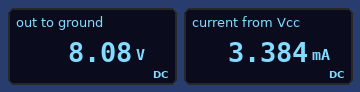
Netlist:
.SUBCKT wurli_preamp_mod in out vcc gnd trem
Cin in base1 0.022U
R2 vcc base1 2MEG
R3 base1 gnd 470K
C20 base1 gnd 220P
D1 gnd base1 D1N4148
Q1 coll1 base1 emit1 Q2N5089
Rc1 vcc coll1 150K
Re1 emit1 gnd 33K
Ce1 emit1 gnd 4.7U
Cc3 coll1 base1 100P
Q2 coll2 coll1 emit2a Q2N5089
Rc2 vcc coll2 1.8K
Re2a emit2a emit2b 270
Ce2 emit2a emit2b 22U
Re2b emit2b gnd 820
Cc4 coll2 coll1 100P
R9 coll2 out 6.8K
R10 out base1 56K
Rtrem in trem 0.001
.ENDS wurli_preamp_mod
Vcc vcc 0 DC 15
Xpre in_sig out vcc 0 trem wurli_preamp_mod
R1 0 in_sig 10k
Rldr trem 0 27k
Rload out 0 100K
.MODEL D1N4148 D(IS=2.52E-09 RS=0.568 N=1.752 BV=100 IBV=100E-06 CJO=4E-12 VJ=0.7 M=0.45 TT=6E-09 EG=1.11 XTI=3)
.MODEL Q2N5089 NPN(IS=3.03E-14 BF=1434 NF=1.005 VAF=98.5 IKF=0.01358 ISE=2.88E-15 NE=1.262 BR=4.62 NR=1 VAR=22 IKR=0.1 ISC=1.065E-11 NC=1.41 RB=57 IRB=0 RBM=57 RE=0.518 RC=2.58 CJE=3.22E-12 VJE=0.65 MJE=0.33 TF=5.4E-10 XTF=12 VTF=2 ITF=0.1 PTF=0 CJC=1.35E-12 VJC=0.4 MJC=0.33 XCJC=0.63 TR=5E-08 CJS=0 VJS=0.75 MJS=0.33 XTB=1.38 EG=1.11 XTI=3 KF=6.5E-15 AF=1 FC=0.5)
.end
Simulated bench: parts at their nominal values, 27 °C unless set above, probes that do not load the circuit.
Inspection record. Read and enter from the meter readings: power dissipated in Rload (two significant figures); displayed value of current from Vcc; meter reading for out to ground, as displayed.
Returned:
650 µW
3.384 mA
8.08 V
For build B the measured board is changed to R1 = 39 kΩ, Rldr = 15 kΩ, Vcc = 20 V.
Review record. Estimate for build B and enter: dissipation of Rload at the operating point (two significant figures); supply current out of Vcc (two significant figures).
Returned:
1.1 mW
4.7 mA
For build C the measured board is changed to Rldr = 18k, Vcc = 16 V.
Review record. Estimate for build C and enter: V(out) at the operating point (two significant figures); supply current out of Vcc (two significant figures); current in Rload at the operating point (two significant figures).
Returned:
8.6 V
3.6 mA
86 µA
